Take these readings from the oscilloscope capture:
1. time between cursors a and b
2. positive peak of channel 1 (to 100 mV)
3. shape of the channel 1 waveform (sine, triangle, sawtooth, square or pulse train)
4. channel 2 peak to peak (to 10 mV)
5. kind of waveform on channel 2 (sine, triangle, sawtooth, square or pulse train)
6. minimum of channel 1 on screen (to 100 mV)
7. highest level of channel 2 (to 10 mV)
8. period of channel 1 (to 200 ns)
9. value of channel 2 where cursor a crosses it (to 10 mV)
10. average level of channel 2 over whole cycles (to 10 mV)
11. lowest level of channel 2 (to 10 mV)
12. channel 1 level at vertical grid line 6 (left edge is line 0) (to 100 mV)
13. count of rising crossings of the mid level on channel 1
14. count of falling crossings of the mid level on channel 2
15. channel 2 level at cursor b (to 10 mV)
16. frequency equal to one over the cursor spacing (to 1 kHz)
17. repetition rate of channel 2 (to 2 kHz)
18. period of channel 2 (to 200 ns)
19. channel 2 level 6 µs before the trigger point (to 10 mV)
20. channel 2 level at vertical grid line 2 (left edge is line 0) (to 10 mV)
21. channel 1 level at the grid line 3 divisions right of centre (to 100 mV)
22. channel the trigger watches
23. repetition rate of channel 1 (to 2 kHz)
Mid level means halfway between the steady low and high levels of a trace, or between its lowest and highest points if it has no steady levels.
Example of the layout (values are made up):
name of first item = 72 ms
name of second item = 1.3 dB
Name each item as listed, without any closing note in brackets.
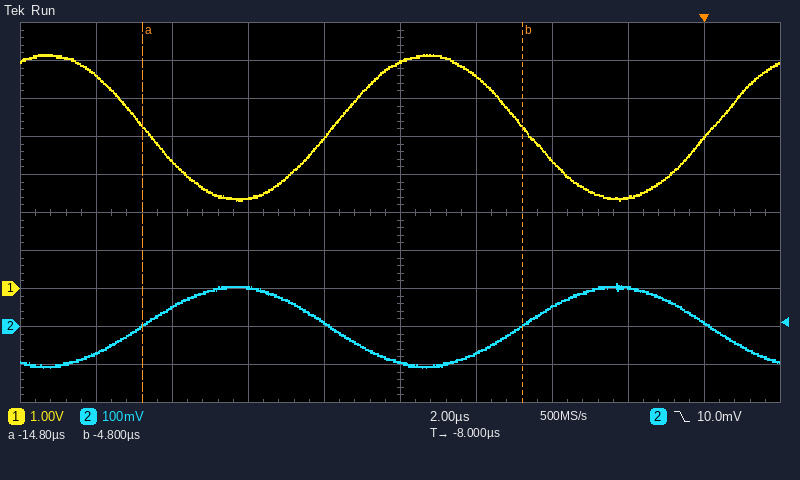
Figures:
time between cursors a and b = 10.0 µs
positive peak of channel 1 = 6.2 V
shape of the channel 1 waveform = sine
channel 2 peak to peak = 220 mV
kind of waveform on channel 2 = sine
minimum of channel 1 on screen = 2.3 V
highest level of channel 2 = 110 mV
period of channel 1 = 10.0 µs
value of channel 2 where cursor a crosses it = 0 mV
average level of channel 2 over whole cycles = 0 mV
lowest level of channel 2 = -110 mV
channel 1 level at vertical grid line 6 (left edge is line 0) = 5.6 V
count of rising crossings of the mid level on channel 1 = 2
count of falling crossings of the mid level on channel 2 = 2
channel 2 level at cursor b = 0 mV
frequency equal to one over the cursor spacing = 100 kHz
repetition rate of channel 2 = 100 kHz
period of channel 2 = 10.0 µs
channel 2 level 6 µs before the trigger point = -70 mV
channel 2 level at vertical grid line 2 (left edge is line 0) = 50 mV
channel 1 level at the grid line 3 divisions right of centre = 2.4 V
channel the trigger watches = channel 2
repetition rate of channel 1 = 100 kHz
